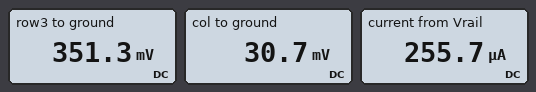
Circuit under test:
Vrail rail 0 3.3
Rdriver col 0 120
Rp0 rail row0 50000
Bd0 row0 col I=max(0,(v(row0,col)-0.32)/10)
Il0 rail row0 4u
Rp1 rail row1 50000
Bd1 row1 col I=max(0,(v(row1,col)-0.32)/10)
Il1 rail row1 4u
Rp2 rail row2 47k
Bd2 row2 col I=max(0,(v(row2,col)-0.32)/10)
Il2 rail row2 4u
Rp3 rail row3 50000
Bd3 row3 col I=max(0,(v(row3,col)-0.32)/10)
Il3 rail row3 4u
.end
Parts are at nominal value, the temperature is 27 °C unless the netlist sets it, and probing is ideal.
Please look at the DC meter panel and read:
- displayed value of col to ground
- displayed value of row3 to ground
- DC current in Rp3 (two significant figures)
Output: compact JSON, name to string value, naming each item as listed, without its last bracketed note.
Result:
{"displayed value of col to ground": "30.7 mV", "displayed value of row3 to ground": "351.3 mV", "DC current in Rp3": "59 µA"}
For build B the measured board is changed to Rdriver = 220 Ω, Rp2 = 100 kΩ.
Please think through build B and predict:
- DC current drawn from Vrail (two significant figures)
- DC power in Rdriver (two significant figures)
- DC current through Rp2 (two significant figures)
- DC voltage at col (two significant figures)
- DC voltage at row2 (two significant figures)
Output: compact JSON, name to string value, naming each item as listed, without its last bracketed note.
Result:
{"DC current drawn from Vrail": "220 µA", "DC power in Rdriver": "11 µW", "DC current through Rp2": "29 µA", "DC voltage at col": "49 mV", "DC voltage at row2": "370 mV"}
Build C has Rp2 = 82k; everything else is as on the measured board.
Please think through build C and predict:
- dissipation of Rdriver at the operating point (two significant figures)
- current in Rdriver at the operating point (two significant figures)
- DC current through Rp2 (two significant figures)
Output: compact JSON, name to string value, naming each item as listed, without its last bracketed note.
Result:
{"dissipation of Rdriver at the operating point": "6.3 µW", "current in Rdriver at the operating point": "230 µA", "DC current through Rp2": "36 µA"}
